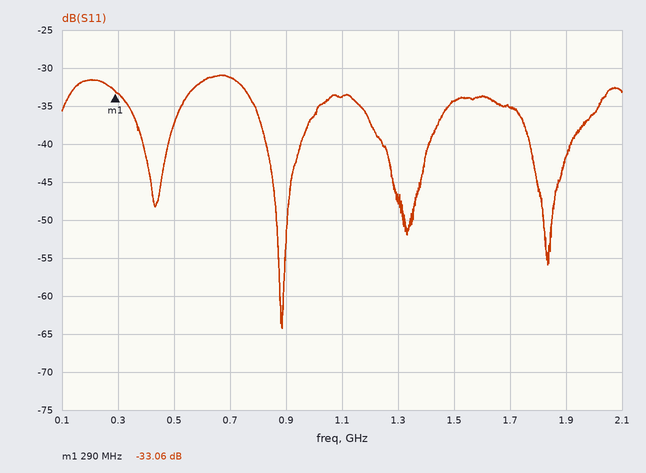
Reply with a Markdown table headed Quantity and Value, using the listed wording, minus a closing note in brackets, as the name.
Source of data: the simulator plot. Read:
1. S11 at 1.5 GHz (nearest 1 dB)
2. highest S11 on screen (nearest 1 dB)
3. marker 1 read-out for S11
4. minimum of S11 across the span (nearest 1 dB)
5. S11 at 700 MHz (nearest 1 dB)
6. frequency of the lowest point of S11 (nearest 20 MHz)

| Quantity | Value |
|---|---|
| S11 at 1.5 GHz | -34 dB |
| highest S11 on screen | -31 dB |
| marker 1 read-out for S11 | -33.06 dB |
| minimum of S11 across the span | -64 dB |
| S11 at 700 MHz | -31 dB |
| frequency of the lowest point of S11 | 880 MHz |
